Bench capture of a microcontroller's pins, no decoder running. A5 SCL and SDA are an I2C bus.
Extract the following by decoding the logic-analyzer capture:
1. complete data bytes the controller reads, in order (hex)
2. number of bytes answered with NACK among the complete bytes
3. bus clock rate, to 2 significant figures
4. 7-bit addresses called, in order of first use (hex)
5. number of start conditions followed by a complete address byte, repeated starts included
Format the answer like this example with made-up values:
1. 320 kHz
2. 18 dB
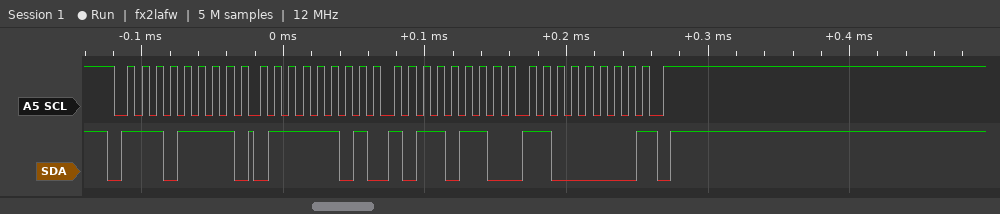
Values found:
1. 7D B6 C0
2. 1
3. 100 kHz
4. 0x77
5. 1
